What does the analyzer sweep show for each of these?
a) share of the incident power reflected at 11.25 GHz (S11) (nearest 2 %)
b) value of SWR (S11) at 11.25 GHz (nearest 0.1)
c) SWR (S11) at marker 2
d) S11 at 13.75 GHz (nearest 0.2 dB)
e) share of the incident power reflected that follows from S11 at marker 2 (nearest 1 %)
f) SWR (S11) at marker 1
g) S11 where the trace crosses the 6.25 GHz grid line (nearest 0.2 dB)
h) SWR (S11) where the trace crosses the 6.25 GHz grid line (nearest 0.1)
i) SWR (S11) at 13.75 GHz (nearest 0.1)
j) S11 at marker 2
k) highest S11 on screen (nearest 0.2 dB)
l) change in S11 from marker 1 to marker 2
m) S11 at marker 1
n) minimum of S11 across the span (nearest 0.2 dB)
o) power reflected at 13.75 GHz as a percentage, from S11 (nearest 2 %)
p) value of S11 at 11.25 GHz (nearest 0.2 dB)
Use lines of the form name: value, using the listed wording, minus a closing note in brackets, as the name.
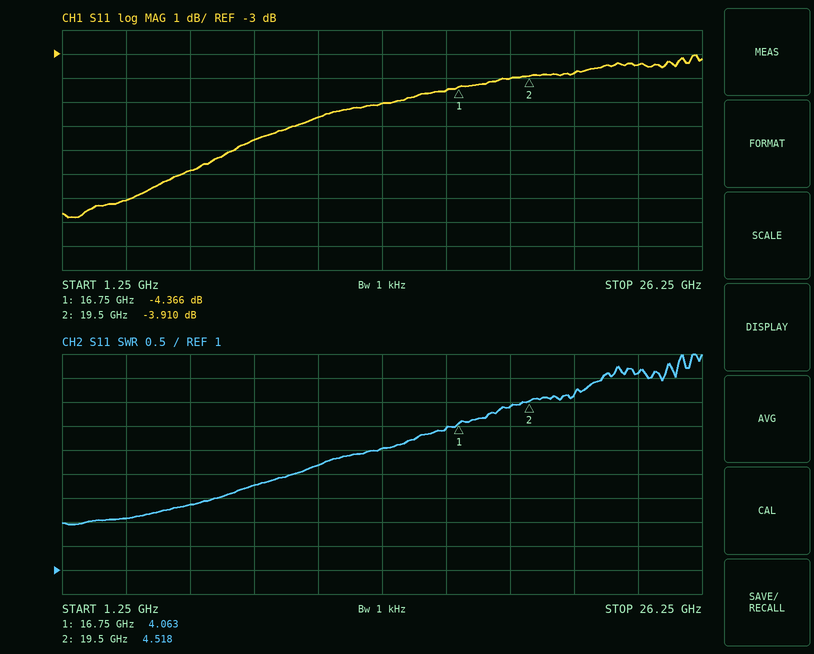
share of the incident power reflected at 11.25 GHz (S11): 28 %
value of SWR (S11) at 11.25 GHz: 3.2
SWR (S11) at marker 2: 4.518
S11 at 13.75 GHz: -5.0 dB
share of the incident power reflected that follows from S11 at marker 2: 41 %
SWR (S11) at marker 1: 4.063
S11 where the trace crosses the 6.25 GHz grid line: -7.8 dB
SWR (S11) where the trace crosses the 6.25 GHz grid line: 2.4
SWR (S11) at 13.75 GHz: 3.5
S11 at marker 2: -3.910 dB
highest S11 on screen: -3.0 dB
change in S11 from marker 1 to marker 2: 0.456 dB
S11 at marker 1: -4.366 dB
minimum of S11 across the span: -9.8 dB
power reflected at 13.75 GHz as a percentage, from S11: 32 %
value of S11 at 11.25 GHz: -5.6 dB
